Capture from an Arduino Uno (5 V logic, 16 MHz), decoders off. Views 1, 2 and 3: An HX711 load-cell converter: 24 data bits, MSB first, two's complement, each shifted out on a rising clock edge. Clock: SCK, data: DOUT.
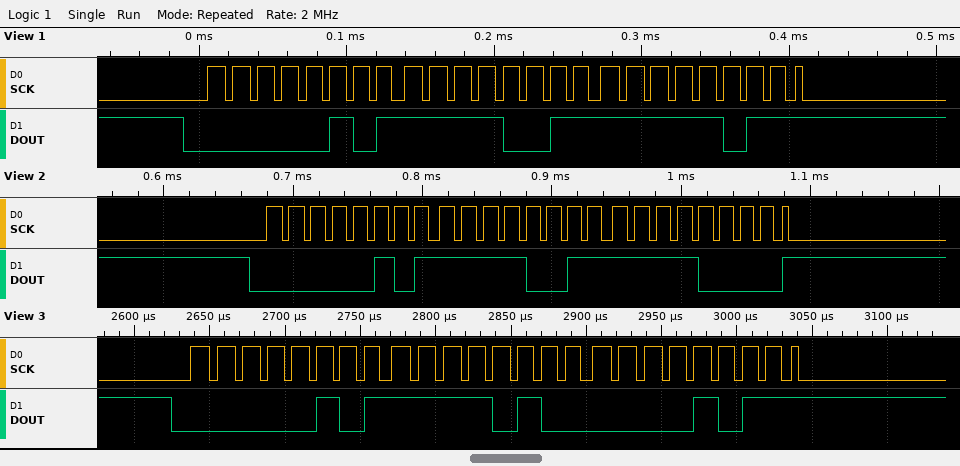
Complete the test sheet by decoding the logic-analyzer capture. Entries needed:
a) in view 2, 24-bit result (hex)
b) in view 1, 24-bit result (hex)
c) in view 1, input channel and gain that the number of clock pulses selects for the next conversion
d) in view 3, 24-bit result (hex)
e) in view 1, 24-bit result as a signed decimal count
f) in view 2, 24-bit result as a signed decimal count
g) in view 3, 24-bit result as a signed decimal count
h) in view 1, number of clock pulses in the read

0x05F3F0
0x05F3FB
channel A, gain 128
0x05F40B
390139
390128
390155
25
